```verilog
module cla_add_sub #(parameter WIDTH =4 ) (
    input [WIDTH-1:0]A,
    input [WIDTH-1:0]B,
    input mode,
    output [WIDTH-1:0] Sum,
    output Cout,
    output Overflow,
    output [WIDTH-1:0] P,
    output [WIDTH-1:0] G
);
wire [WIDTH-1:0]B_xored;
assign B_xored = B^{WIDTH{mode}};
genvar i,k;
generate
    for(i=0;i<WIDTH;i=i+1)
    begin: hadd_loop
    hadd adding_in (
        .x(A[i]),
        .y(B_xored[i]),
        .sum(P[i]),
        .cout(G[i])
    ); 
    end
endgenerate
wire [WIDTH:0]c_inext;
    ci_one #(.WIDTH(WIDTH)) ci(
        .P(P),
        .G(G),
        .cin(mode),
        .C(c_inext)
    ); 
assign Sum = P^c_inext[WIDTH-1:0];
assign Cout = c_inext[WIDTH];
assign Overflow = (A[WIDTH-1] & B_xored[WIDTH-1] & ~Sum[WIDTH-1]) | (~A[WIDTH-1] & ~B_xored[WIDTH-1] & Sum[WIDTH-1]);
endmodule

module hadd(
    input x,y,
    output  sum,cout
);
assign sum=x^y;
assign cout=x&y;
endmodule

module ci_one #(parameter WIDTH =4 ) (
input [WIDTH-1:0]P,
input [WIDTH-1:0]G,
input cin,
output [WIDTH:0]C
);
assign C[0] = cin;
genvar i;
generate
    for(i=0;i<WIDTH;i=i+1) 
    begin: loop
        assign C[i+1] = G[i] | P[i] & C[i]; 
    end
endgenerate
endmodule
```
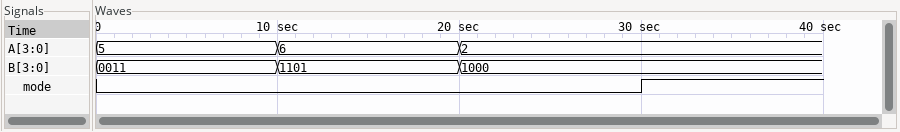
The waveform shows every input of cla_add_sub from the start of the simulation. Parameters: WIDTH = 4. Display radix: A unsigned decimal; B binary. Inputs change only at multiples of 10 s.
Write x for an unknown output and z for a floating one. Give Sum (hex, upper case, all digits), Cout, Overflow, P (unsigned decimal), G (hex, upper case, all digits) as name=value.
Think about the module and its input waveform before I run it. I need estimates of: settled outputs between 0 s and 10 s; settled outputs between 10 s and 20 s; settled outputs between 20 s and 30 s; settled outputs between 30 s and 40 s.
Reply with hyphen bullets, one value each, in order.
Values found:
- Sum=8, Cout=0, Overflow=1, P=6, G=1
- Sum=3, Cout=1, Overflow=0, P=11, G=4
- Sum=A, Cout=0, Overflow=0, P=10, G=0
- Sum=A, Cout=0, Overflow=1, P=5, G=2
